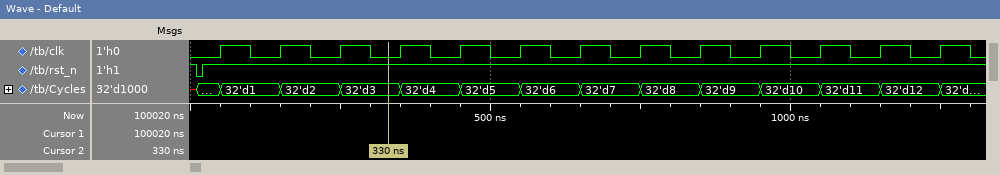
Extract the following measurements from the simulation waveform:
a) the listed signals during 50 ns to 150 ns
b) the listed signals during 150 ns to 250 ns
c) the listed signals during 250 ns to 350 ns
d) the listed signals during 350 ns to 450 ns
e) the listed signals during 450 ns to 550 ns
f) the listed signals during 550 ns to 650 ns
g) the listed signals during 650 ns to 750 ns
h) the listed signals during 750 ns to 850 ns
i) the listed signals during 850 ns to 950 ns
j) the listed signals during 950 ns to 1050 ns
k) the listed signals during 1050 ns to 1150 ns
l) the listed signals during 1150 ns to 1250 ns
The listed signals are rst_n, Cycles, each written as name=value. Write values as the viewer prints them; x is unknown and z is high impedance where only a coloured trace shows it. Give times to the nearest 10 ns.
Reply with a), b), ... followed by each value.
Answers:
a) rst_n=1, Cycles=32'd1
b) rst_n=1, Cycles=32'd2
c) rst_n=1, Cycles=32'd3
d) rst_n=1, Cycles=32'd4
e) rst_n=1, Cycles=32'd5
f) rst_n=1, Cycles=32'd6
g) rst_n=1, Cycles=32'd7
h) rst_n=1, Cycles=32'd8
i) rst_n=1, Cycles=32'd9
j) rst_n=1, Cycles=32'd10
k) rst_n=1, Cycles=32'd11
l) rst_n=1, Cycles=32'd12
